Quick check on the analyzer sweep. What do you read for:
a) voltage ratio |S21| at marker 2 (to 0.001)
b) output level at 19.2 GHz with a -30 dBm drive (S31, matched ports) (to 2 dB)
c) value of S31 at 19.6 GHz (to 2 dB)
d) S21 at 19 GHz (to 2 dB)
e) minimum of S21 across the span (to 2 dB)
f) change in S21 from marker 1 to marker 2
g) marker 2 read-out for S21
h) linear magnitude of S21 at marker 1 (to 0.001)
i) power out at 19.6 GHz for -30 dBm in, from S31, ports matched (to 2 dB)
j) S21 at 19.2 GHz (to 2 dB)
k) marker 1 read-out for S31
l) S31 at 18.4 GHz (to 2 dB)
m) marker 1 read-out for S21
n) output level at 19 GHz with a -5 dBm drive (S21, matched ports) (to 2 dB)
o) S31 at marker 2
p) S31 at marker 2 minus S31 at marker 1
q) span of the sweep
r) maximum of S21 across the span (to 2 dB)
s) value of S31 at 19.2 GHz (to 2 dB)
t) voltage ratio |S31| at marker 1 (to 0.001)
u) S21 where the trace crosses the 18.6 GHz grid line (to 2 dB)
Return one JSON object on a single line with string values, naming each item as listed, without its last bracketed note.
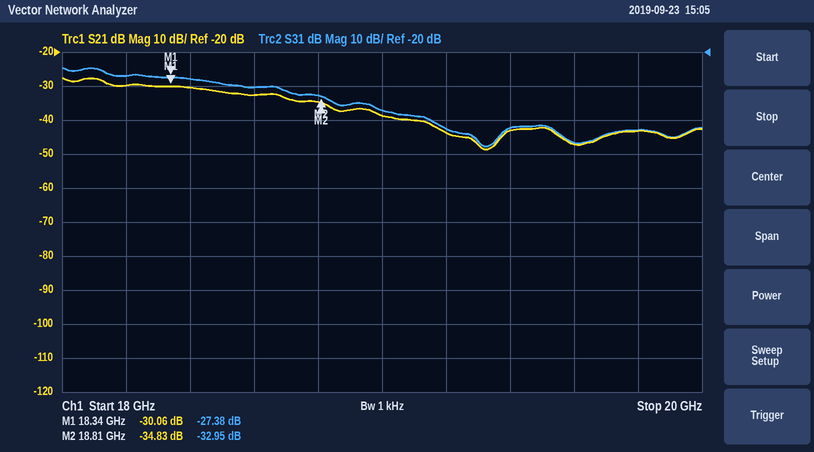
{"voltage ratio |S21| at marker 2": "0.018", "output level at 19.2 GHz with a -30 dBm drive (S31, matched ports)": "-72 dBm", "value of S31 at 19.6 GHz": "-46 dB", "S21 at 19 GHz": "-38 dB", "minimum of S21 across the span": "-48 dB", "change in S21 from marker 1 to marker 2": "-4.77 dB", "marker 2 read-out for S21": "-34.83 dB", "linear magnitude of S21 at marker 1": "0.031", "power out at 19.6 GHz for -30 dBm in, from S31, ports matched": "-76 dBm", "S21 at 19.2 GHz": "-44 dB", "marker 1 read-out for S31": "-27.38 dB", "S31 at 18.4 GHz": "-28 dB", "marker 1 read-out for S21": "-30.06 dB", "output level at 19 GHz with a -5 dBm drive (S21, matched ports)": "-44 dBm", "S31 at marker 2": "-32.95 dB", "S31 at marker 2 minus S31 at marker 1": "-5.57 dB", "span of the sweep": "2 GHz", "maximum of S21 across the span": "-28 dB", "value of S31 at 19.2 GHz": "-42 dB", "voltage ratio |S31| at marker 1": "0.043", "S21 where the trace crosses the 18.6 GHz grid line": "-32 dB"}
